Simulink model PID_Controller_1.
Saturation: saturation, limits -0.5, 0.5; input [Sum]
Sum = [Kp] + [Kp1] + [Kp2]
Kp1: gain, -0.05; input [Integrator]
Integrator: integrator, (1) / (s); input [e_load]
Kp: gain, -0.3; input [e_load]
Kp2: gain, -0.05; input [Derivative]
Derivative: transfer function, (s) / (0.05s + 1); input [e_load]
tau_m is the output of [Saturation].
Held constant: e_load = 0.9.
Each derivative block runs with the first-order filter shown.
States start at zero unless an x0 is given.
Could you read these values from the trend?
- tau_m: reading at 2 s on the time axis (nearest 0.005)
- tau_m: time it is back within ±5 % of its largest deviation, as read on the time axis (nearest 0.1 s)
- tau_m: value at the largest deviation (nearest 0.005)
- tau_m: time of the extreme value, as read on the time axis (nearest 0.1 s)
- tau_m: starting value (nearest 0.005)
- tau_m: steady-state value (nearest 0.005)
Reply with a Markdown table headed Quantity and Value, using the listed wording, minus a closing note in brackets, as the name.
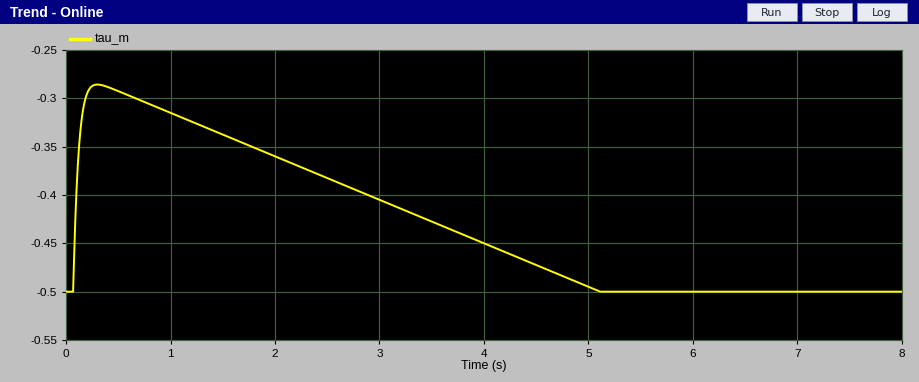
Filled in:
| Quantity | Value |
|---|---|
| tau_m: reading at 2 s on the time axis | -0.360 |
| tau_m: time it is back within ±5 % of its largest deviation, as read on the time axis | 4.9 s |
| tau_m: value at the largest deviation | -0.285 |
| tau_m: time of the extreme value, as read on the time axis | 0.3 s |
| tau_m: starting value | -0.500 |
| tau_m: steady-state value | -0.500 |
